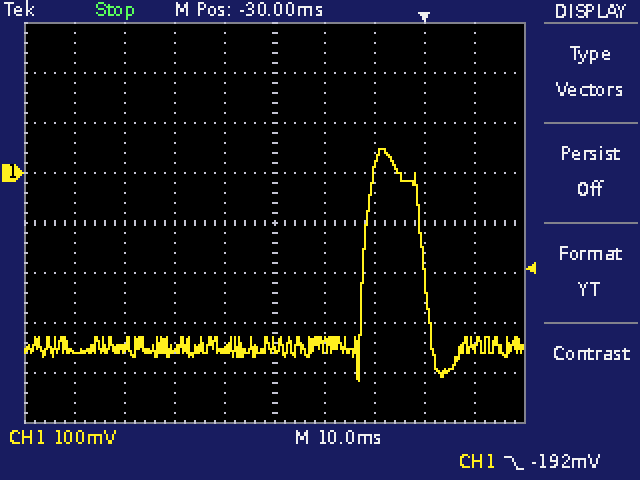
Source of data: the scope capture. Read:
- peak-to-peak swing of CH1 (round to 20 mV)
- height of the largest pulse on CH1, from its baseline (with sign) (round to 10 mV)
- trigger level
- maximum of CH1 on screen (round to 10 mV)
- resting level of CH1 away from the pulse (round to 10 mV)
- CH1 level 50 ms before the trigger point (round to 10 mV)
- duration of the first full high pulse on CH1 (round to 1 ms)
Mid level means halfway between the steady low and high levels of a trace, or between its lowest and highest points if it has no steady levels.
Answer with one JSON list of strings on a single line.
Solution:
["460 mV", "+400 mV", "-192 mV", "50 mV", "-350 mV", "-350 mV", "12 ms"]
